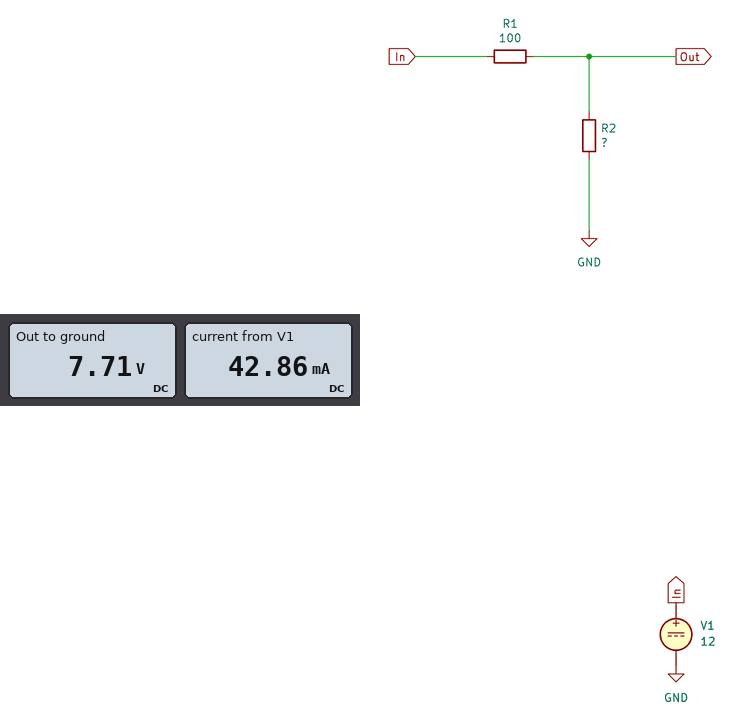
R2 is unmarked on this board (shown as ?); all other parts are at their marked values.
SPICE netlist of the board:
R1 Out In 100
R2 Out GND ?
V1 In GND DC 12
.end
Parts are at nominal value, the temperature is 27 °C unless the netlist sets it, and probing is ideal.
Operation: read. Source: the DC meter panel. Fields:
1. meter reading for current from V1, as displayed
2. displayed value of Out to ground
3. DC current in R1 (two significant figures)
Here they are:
42.86 mA
7.71 V
43 mA
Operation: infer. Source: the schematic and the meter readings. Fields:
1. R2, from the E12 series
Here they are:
180 Ω
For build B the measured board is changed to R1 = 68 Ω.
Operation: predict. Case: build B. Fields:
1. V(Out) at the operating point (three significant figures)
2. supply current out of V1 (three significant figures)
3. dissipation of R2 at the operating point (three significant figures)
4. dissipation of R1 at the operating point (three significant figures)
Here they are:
8.71 V
48.4 mA
421 mW
159 mW
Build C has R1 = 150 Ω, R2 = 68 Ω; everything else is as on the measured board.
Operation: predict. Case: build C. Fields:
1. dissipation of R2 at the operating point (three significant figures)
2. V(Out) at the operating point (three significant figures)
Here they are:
206 mW
3.74 V
